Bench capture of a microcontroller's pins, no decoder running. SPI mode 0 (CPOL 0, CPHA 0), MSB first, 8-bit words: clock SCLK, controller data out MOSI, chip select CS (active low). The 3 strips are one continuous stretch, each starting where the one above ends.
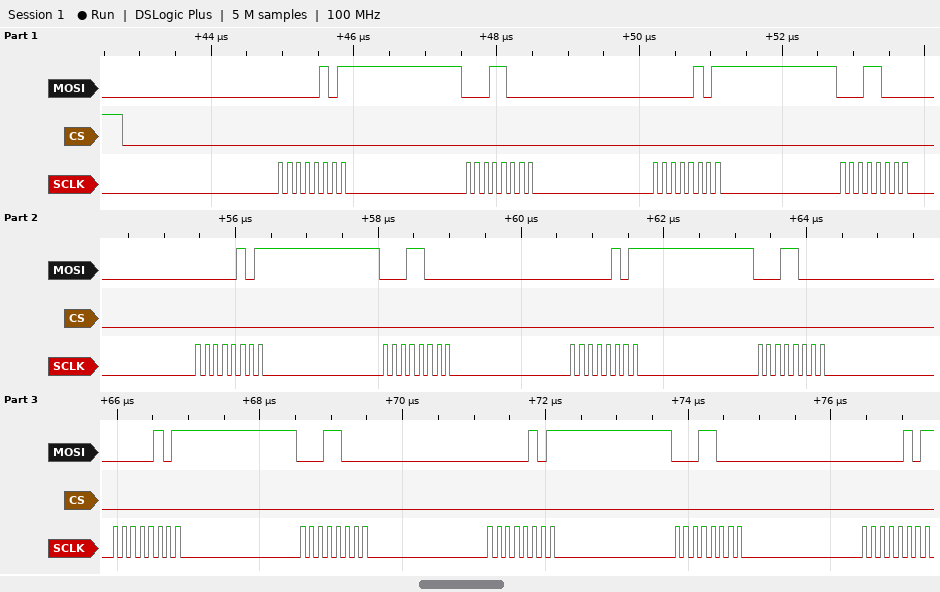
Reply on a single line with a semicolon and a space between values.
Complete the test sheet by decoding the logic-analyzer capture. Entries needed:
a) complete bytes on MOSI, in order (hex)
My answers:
0x05 0x18 0x05 0x18 0x05 0x18 0x05 0x18 0x05 0x18 0x05 0x18 0x05
